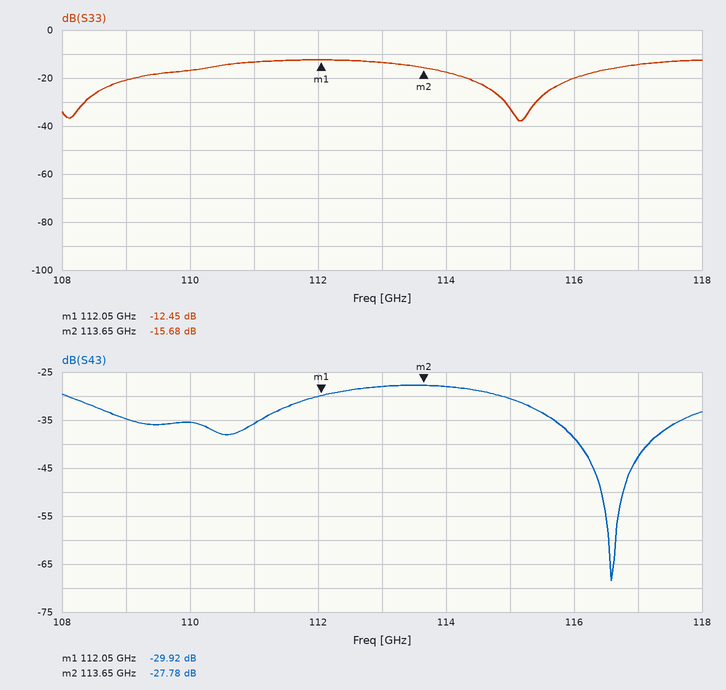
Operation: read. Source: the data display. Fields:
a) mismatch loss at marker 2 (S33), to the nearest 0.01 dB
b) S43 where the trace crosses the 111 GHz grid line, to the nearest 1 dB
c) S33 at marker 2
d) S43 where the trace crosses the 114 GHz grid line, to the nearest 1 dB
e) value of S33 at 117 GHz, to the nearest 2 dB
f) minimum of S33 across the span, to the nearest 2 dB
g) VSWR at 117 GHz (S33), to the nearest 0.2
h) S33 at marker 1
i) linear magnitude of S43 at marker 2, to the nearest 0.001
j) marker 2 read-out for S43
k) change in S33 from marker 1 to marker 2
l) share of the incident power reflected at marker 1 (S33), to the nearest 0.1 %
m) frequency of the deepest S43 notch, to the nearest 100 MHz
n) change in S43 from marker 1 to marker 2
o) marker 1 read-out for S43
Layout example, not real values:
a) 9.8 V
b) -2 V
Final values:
a) 0.12 dB
b) -36 dB
c) -15.68 dB
d) -28 dB
e) -14 dB
f) -38 dB
g) 1.4
h) -12.45 dB
i) 0.041
j) -27.78 dB
k) -3.23 dB
l) 5.7 %
m) 116.6 GHz
n) 2.14 dB
o) -29.92 dB
